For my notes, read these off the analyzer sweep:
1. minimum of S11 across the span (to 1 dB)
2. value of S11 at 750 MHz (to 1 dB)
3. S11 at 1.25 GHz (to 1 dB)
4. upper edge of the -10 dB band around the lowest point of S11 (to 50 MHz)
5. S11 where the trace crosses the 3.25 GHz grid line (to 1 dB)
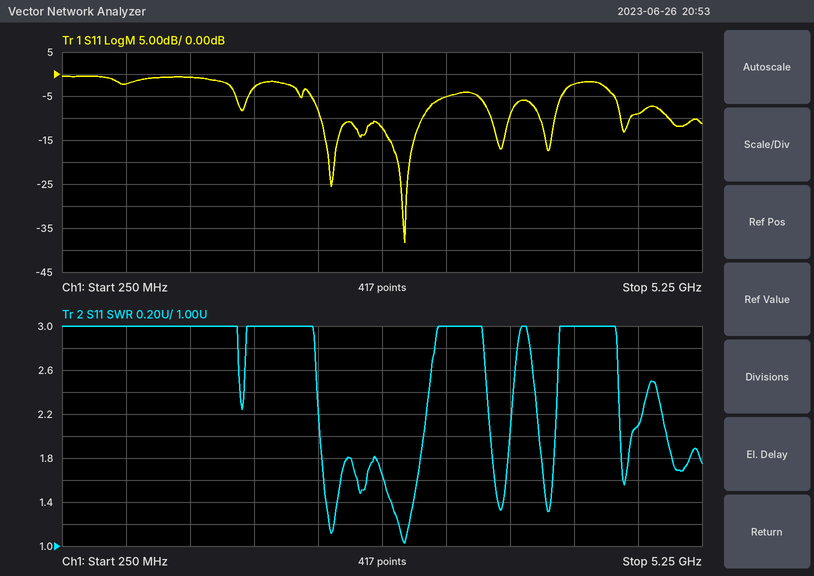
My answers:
-38 dB
-2 dB
-1 dB
3.05 GHz
-5 dB
